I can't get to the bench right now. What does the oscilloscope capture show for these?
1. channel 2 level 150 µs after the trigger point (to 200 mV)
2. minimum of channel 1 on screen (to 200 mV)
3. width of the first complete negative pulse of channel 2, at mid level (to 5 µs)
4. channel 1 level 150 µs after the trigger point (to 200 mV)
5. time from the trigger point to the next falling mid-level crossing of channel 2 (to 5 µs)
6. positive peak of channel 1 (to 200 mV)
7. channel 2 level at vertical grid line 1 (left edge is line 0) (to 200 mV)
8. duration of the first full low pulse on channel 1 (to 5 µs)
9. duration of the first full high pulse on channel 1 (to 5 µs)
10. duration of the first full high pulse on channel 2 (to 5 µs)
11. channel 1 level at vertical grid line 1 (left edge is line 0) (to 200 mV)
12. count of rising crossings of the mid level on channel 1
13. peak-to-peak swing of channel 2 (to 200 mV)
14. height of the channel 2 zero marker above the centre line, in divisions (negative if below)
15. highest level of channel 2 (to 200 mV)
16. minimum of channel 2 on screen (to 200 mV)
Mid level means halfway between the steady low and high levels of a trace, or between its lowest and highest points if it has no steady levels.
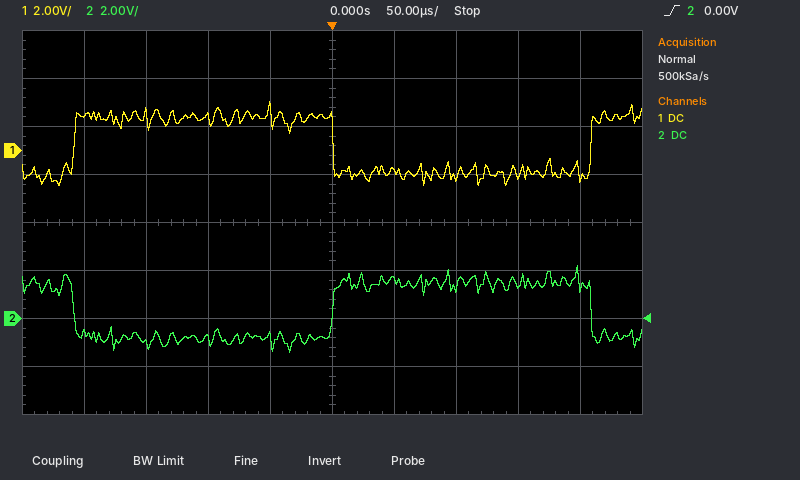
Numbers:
1.4 V
-1.4 V
210 µs
-1.0 V
210 µs
2.0 V
-600 mV
210 µs
210 µs
210 µs
1.4 V
2
3.6 V
-2.0 div
2.2 V
-1.4 V
